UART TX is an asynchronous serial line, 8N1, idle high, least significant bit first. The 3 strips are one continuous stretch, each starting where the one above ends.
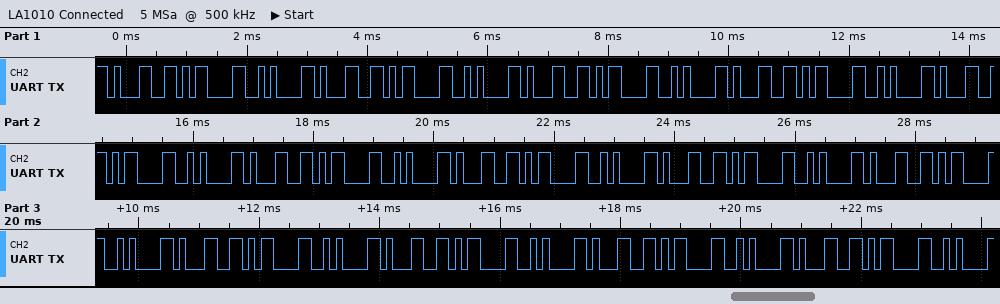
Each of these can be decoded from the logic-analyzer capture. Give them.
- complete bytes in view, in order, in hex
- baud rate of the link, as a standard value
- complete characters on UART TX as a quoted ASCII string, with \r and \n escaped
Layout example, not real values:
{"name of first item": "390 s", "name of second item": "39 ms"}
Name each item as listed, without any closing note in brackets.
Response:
{"complete bytes in view, in order, in hex": "0x31 0x0D 0x0A 0x31 0x0D 0x0A 0x31 0x0D 0x0A 0x31 0x0D 0x0A 0x31 0x0D 0x0A 0x31 0x0D 0x0A 0x31 0x0D 0x0A 0x31 0x0D 0x0A 0x31 0x0D 0x0A 0x31 0x0D 0x0A 0x31 0x0D 0x0A 0x31 0x0D 0x0A 0x31 0x0D 0x0A", "baud rate of the link, as a standard value": "9600 baud", "complete characters on UART TX as a quoted ASCII string, with \\r and \\n escaped": "\"1\\r\\n1\\r\\n1\\r\\n1\\r\\n1\\r\\n1\\r\\n1\\r\\n1\\r\\n1\\r\\n1\\r\\n1\\r\\n1\\r\\n1\\r\\n\""}
